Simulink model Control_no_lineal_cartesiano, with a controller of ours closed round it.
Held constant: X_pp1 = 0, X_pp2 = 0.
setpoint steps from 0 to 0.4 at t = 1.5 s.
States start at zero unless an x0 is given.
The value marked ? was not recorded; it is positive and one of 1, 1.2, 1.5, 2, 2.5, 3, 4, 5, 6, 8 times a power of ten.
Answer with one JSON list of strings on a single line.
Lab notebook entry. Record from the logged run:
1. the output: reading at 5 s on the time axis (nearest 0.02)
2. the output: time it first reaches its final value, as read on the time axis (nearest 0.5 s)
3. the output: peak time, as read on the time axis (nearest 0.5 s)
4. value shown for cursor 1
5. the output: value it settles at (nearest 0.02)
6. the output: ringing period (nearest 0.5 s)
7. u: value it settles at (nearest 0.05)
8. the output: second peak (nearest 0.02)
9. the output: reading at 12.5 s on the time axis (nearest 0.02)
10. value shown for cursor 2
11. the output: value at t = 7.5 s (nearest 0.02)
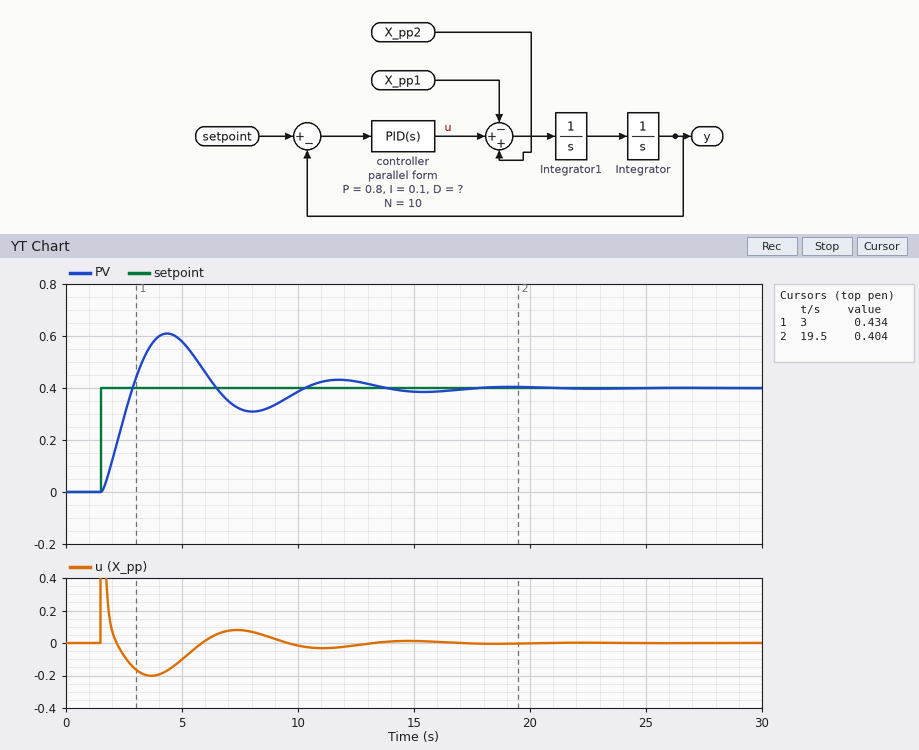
["0.58", "3.0 s", "4.5 s", "0.434", "0.40", "7.5 s", "0.00", "0.44", "0.42", "0.404", "0.32"]
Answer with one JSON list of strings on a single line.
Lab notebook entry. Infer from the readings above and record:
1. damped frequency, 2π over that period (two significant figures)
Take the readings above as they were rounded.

["0.84 rad/s"]
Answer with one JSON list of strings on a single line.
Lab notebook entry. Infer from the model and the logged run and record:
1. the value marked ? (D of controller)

["0.6"]
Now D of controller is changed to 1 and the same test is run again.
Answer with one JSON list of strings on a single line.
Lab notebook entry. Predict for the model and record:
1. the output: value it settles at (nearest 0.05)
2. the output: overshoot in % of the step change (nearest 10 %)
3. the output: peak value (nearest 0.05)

["0.40", "30 %", "0.55"]
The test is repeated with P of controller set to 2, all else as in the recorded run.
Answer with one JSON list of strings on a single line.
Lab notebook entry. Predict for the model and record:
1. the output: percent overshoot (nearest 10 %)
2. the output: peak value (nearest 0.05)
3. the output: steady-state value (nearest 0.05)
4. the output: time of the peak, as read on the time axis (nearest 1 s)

["60 %", "0.65", "0.40", "3 s"]
